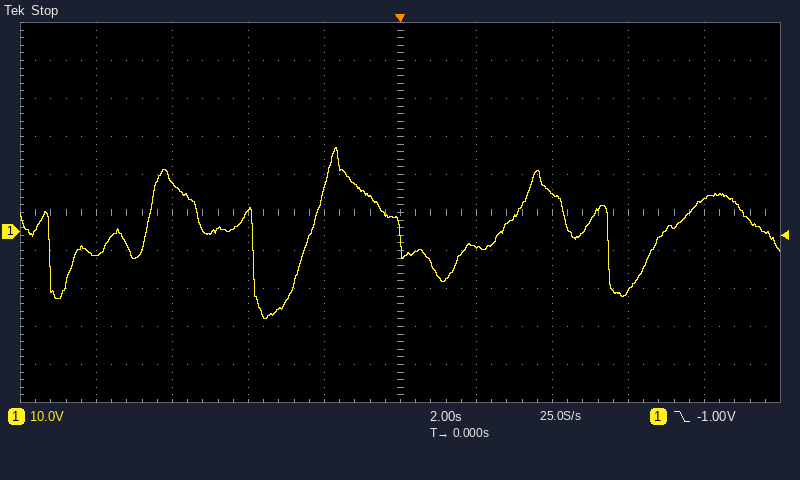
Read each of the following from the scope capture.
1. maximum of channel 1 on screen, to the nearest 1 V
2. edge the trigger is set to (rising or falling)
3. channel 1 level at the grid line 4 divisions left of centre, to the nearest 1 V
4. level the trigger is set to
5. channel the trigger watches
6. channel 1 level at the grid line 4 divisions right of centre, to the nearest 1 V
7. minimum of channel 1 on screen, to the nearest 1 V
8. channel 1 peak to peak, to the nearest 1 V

22 V
falling
-6 V
-1.00 V
channel 1
9 V
-23 V
45 V
